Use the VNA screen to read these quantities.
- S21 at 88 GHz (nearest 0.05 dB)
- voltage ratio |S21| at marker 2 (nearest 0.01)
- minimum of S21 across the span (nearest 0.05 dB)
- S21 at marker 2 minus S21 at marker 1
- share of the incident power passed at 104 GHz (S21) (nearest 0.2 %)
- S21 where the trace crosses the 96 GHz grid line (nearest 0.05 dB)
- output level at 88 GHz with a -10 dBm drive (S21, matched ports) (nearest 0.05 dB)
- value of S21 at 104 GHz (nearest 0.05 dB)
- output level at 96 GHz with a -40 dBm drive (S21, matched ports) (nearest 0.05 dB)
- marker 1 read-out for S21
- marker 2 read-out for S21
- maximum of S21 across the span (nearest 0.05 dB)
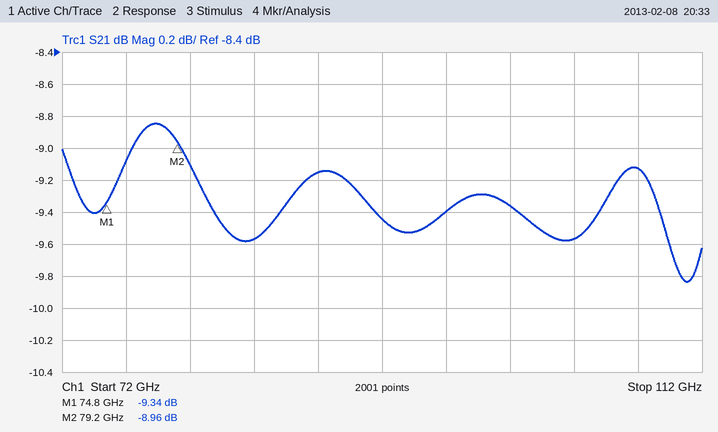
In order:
-9.15 dB
0.36
-9.85 dB
0.38 dB
11.0 %
-9.40 dB
-19.15 dBm
-9.55 dB
-49.40 dBm
-9.34 dB
-8.96 dB
-8.85 dB
